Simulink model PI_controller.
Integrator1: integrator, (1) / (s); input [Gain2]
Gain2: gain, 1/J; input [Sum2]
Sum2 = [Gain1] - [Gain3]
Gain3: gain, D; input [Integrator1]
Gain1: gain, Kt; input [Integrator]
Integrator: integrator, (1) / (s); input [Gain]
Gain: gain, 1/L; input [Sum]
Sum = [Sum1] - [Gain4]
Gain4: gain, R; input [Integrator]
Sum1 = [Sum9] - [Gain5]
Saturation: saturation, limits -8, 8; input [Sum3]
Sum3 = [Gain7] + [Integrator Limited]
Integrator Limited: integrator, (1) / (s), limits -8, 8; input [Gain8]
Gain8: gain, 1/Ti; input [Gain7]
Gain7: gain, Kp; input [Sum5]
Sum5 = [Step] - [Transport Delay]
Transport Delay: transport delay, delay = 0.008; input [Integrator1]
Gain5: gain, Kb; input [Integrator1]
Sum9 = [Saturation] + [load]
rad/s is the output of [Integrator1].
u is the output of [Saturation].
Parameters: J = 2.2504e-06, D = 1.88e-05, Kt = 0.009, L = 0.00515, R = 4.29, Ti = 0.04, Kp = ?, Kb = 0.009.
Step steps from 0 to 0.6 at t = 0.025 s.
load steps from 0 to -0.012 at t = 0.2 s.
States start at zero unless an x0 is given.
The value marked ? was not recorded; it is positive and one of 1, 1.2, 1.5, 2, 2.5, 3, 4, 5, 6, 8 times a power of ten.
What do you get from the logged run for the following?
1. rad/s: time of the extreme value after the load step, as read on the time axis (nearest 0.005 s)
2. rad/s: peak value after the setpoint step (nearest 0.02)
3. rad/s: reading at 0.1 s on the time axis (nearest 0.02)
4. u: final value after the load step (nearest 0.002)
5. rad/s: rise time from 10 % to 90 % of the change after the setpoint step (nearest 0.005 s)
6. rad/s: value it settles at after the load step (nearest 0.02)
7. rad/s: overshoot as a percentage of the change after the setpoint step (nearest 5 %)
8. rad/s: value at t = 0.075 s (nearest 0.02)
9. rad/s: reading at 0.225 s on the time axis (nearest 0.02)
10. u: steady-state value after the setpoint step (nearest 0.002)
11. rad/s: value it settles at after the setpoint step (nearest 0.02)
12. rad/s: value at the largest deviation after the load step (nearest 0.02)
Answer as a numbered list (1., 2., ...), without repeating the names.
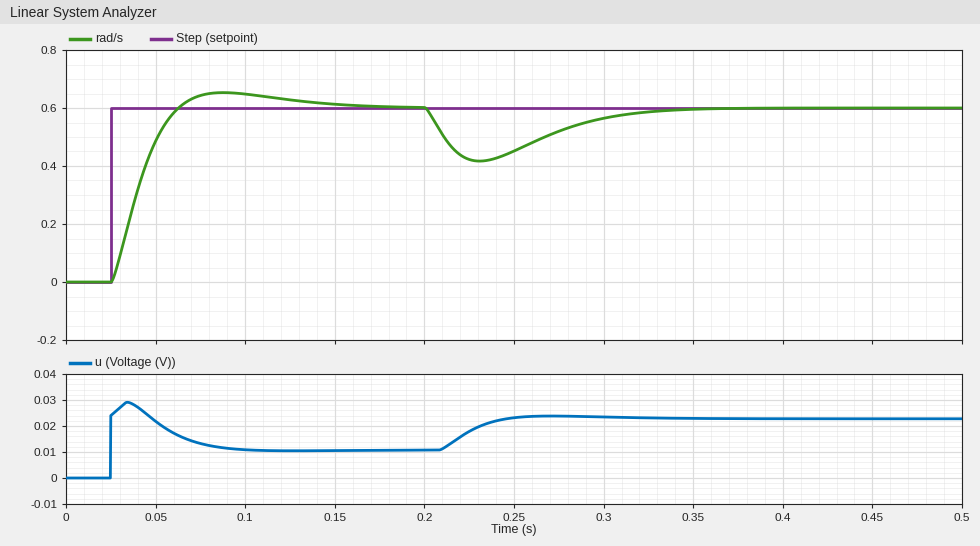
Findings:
1. 0.230 s
2. 0.66
3. 0.64
4. 0.022
5. 0.025 s
6. 0.60
7. 10 %
8. 0.64
9. 0.42
10. 0.010
11. 0.60
12. 0.42
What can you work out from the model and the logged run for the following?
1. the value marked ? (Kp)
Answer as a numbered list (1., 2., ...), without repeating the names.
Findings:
1. 0.04
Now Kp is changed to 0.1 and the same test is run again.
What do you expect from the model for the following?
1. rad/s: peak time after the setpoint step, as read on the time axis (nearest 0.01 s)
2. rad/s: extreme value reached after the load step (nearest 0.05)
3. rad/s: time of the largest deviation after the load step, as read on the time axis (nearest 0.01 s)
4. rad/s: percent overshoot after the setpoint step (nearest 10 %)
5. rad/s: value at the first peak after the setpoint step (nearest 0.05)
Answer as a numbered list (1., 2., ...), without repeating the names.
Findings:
1. 0.05 s
2. 0.45
3. 0.22 s
4. 50 %
5. 0.90
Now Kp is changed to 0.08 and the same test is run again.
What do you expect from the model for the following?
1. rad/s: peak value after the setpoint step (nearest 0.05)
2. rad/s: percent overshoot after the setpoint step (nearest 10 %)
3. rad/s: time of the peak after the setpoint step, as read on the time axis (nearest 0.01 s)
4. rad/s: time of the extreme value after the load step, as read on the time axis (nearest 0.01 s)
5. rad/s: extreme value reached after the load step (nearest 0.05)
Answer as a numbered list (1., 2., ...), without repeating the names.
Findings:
1. 0.80
2. 30 %
3. 0.05 s
4. 0.22 s
5. 0.45
